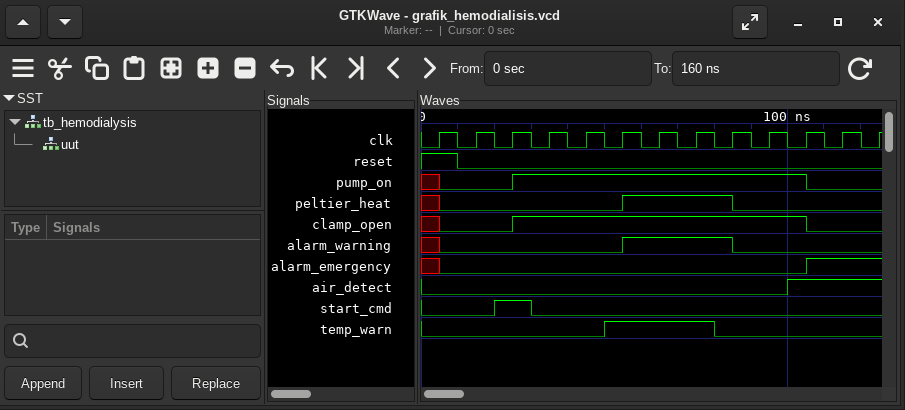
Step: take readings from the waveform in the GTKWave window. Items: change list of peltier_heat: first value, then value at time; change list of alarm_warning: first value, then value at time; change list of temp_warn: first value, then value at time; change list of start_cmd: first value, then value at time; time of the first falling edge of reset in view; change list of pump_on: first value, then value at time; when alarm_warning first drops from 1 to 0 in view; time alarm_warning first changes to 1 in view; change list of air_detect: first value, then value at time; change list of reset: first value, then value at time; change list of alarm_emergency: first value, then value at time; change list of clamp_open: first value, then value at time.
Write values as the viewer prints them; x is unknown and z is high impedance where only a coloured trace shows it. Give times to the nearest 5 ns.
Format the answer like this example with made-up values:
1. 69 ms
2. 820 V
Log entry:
1. x, 0 at 5 ns, 1 at 55 ns, 0 at 85 ns
2. x, 0 at 5 ns, 1 at 55 ns, 0 at 85 ns
3. 0, 1 at 50 ns, 0 at 80 ns
4. 0, 1 at 20 ns, 0 at 30 ns
5. 10 ns
6. x, 0 at 5 ns, 1 at 25 ns, 0 at 105 ns
7. 85 ns
8. 55 ns
9. 0, 1 at 100 ns
10. 1, 0 at 10 ns
11. x, 0 at 5 ns, 1 at 105 ns
12. x, 0 at 5 ns, 1 at 25 ns, 0 at 105 ns
